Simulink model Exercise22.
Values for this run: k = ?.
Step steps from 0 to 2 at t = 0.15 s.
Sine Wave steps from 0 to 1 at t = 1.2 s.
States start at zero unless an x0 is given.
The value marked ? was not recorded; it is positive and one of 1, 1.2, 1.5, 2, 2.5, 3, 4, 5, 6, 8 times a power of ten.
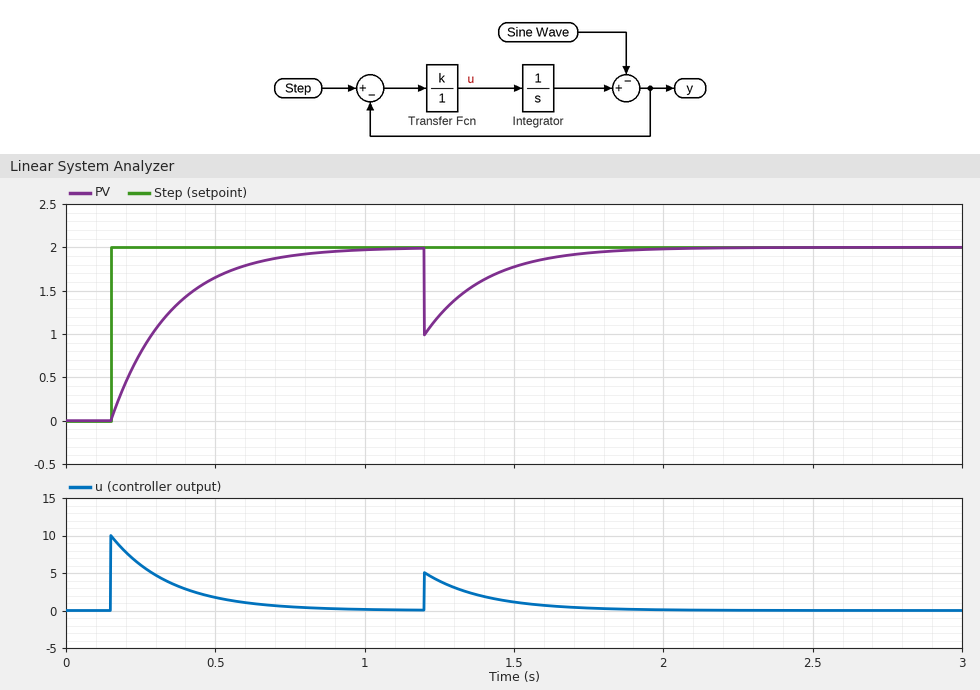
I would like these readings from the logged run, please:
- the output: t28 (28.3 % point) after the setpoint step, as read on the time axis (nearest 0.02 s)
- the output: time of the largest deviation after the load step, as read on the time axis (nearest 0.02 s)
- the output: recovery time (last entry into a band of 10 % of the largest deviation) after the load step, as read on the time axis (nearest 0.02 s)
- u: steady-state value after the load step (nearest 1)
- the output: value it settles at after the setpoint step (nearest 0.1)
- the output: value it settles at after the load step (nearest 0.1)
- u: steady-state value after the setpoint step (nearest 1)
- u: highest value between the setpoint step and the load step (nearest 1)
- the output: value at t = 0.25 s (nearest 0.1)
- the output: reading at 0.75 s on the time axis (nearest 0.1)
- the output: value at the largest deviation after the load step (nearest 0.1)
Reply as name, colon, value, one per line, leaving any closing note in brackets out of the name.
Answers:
the output: t28 (28.3 % point) after the setpoint step, as read on the time axis: 0.22 s
the output: time of the largest deviation after the load step, as read on the time axis: 1.20 s
the output: recovery time (last entry into a band of 10 % of the largest deviation) after the load step, as read on the time axis: 1.66 s
u: steady-state value after the load step: 0
the output: value it settles at after the setpoint step: 2.0
the output: value it settles at after the load step: 2.0
u: steady-state value after the setpoint step: 0
u: highest value between the setpoint step and the load step: 10
the output: value at t = 0.25 s: 0.8
the output: reading at 0.75 s on the time axis: 1.9
the output: value at the largest deviation after the load step: 1.0
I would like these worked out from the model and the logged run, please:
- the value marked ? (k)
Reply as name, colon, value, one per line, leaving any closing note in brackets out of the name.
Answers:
the value marked ?: 5
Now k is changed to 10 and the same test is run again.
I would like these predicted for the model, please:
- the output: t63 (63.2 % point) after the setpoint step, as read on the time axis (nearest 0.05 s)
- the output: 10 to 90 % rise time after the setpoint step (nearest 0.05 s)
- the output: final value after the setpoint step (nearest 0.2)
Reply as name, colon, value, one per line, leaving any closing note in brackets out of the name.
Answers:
the output: t63 (63.2 % point) after the setpoint step, as read on the time axis: 0.25 s
the output: 10 to 90 % rise time after the setpoint step: 0.20 s
the output: final value after the setpoint step: 2.0
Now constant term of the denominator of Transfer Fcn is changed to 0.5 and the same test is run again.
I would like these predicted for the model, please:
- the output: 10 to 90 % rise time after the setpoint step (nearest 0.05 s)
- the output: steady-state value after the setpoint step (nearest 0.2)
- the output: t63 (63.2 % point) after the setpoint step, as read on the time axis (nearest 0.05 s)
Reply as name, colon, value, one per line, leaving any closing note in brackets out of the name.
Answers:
the output: 10 to 90 % rise time after the setpoint step: 0.20 s
the output: steady-state value after the setpoint step: 2.0
the output: t63 (63.2 % point) after the setpoint step, as read on the time axis: 0.25 s
